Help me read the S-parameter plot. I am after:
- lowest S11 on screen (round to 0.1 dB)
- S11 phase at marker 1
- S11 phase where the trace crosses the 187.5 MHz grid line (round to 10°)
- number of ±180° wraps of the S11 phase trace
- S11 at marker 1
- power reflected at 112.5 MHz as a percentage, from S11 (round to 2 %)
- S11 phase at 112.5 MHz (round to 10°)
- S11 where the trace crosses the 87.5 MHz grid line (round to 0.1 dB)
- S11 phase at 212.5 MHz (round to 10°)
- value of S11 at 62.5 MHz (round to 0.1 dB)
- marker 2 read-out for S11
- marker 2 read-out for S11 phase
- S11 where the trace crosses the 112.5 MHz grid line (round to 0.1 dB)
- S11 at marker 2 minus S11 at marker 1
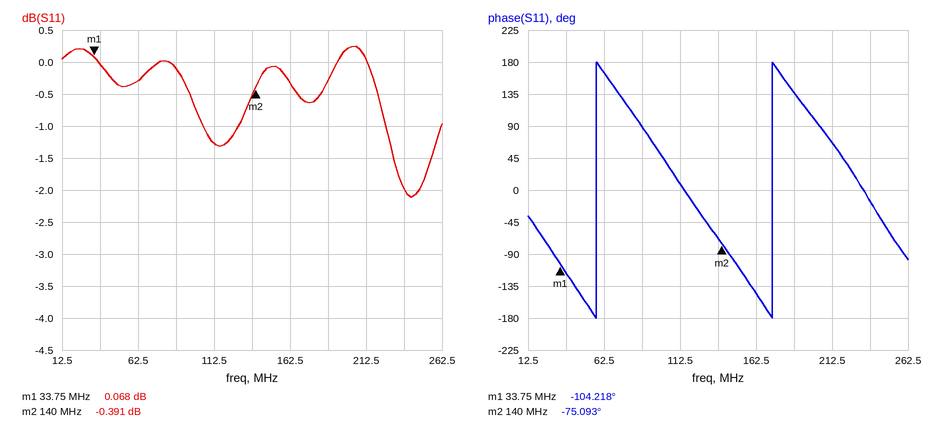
-2.1 dB
-104.218°
140°
2
0.068 dB
74 %
10°
-0.1 dB
70°
-0.3 dB
-0.391 dB
-75.093°
-1.3 dB
-0.459 dB
